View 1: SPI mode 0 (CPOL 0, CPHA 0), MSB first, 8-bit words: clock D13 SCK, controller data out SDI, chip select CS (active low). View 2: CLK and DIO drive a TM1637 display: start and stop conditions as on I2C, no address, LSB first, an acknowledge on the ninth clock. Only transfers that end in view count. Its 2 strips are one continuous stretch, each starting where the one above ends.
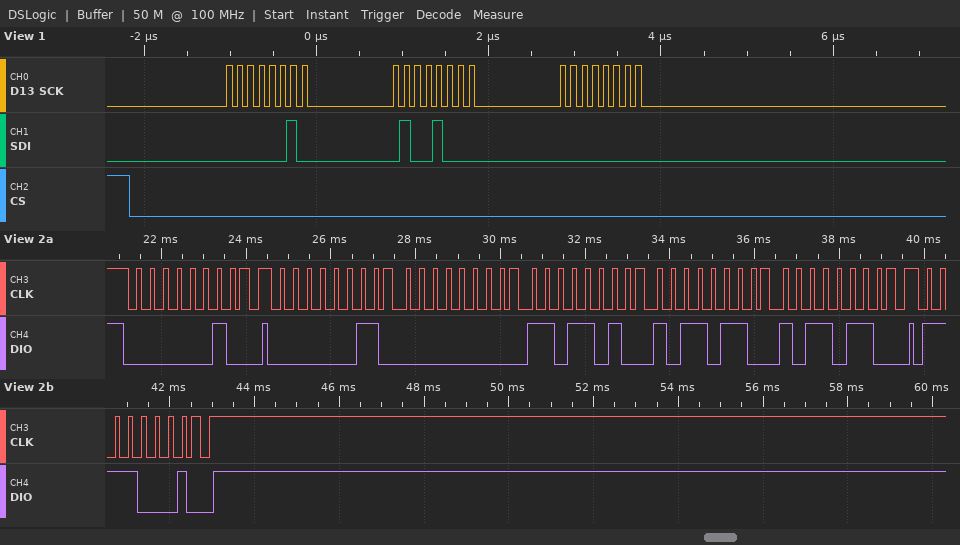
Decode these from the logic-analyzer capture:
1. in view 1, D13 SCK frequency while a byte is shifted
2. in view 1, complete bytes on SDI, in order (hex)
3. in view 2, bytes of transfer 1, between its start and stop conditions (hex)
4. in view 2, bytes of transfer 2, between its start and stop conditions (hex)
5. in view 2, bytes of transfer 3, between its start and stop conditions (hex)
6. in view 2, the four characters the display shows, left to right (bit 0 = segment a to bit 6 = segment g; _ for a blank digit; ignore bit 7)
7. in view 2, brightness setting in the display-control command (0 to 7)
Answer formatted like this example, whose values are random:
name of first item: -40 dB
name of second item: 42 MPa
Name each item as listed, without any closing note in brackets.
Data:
in view 1, D13 SCK frequency while a byte is shifted: 8 MHz
in view 1, complete bytes on SDI, in order: 02 48 00
in view 2, bytes of transfer 1, between its start and stop conditions: 40
in view 2, bytes of transfer 2, between its start and stop conditions: C0 00 5B 6D 6D
in view 2, bytes of transfer 3, between its start and stop conditions: 8F
in view 2, the four characters the display shows, left to right: _255
in view 2, brightness setting in the display-control command: 7
